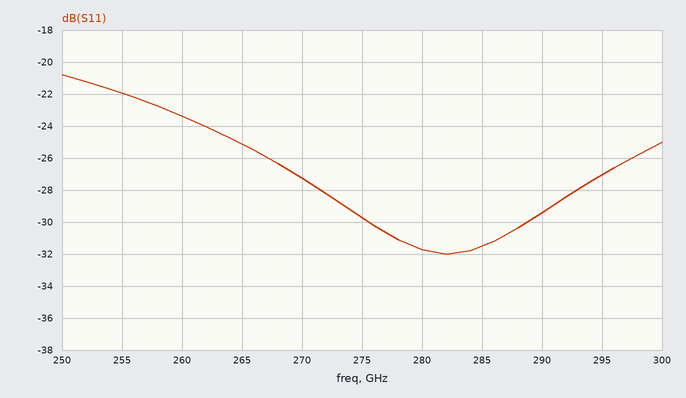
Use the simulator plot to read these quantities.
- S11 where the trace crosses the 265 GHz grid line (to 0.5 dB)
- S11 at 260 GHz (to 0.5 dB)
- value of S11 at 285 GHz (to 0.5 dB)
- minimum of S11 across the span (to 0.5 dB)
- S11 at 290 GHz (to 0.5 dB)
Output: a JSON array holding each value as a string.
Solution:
["-25.0 dB", "-23.5 dB", "-31.5 dB", "-32.0 dB", "-29.5 dB"]
